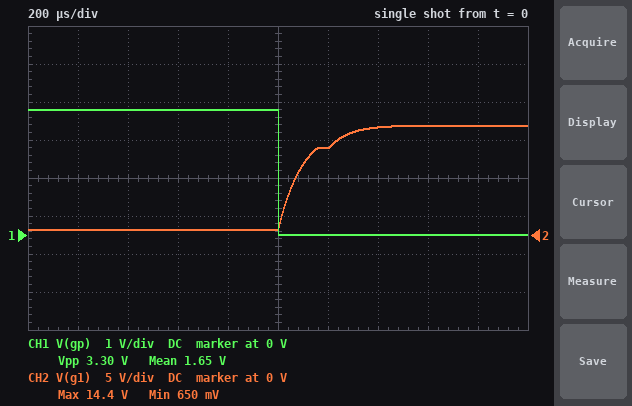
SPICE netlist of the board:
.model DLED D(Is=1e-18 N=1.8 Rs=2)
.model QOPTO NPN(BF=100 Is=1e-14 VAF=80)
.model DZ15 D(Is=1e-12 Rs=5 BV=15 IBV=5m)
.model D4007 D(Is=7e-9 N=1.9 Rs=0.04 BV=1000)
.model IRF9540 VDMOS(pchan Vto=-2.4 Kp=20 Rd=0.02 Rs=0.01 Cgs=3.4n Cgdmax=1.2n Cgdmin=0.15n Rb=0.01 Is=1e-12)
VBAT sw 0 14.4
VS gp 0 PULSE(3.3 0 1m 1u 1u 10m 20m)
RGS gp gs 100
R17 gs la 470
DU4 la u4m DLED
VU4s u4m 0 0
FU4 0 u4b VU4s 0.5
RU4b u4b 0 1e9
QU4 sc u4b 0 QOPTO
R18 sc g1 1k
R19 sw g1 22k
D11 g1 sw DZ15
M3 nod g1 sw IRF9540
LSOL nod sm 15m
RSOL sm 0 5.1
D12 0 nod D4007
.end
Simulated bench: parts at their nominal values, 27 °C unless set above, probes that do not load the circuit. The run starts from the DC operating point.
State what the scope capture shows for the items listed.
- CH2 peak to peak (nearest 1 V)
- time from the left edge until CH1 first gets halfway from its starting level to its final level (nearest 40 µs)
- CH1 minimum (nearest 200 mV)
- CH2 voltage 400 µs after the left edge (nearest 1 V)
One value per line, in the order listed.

14 V
1.00 ms
0 V
1 V
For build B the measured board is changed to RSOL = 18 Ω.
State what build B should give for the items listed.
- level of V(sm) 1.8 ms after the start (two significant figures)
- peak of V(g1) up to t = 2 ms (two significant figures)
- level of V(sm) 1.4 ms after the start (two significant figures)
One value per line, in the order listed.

6.5 V
14 V
11 V
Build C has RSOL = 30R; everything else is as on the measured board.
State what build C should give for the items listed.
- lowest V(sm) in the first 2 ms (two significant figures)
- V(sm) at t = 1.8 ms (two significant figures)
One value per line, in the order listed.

2.3 V
3.8 V
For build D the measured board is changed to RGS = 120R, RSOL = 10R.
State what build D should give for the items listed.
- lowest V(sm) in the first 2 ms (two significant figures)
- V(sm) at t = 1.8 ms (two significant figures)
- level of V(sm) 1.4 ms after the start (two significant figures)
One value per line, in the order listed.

8.0 V
9.3 V
12 V
